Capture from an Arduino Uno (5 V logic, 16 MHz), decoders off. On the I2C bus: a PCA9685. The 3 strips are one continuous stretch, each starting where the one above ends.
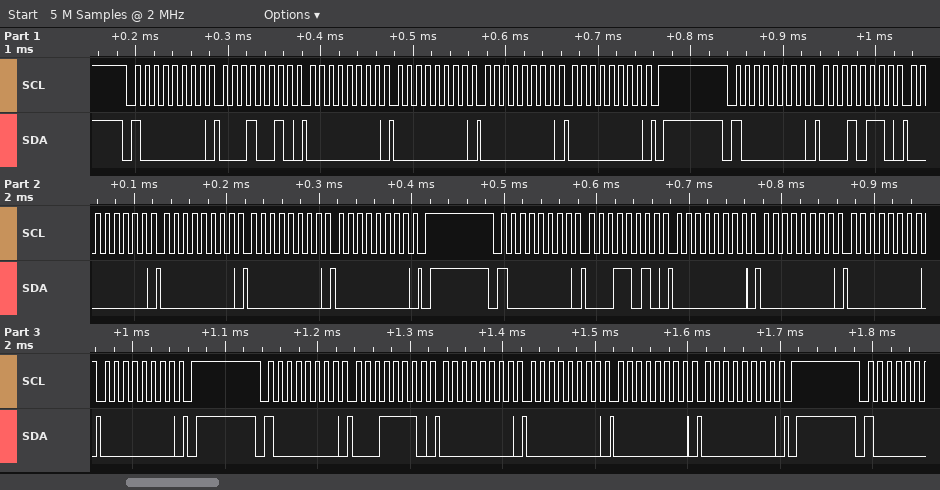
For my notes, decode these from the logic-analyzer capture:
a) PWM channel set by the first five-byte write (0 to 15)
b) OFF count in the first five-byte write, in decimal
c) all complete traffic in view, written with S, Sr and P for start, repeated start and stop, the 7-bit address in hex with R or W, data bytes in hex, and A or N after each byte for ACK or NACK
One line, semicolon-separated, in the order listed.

3; 0; S 40W A 12 A 00 A 00 A 00 A 00 A P S 40W A 16 A 00 A 00 A 00 A 00 A P S 40W A 1A A 00 A 00 A 00 A 00 A P S 40W A 1E A 00 A 00 A 00 A 00 A P
